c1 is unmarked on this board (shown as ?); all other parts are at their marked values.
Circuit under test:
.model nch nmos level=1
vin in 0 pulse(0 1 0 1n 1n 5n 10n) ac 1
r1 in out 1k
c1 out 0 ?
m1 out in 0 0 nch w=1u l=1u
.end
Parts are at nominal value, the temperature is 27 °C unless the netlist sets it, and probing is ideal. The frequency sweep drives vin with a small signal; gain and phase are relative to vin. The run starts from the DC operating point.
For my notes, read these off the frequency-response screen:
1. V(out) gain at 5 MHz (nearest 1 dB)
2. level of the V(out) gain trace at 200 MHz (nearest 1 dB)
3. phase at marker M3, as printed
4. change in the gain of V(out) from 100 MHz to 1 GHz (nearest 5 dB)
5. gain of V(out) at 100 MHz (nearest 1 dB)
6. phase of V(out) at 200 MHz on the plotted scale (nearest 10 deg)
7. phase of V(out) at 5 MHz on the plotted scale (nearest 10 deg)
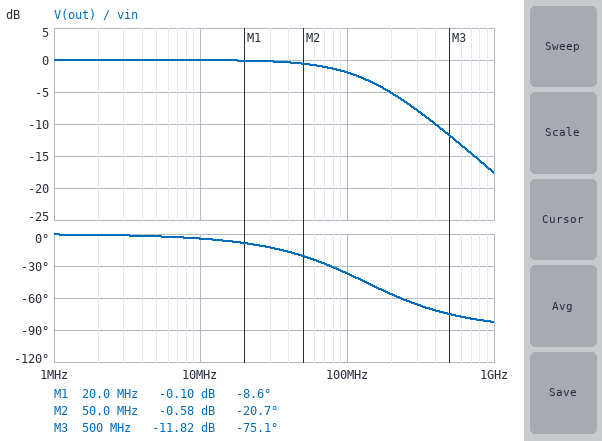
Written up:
0 dB
-5 dB
-75.1 deg
-15 dB
-2 dB
-60 deg
0 deg
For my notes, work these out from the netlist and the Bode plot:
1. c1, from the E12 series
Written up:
1.2 pF
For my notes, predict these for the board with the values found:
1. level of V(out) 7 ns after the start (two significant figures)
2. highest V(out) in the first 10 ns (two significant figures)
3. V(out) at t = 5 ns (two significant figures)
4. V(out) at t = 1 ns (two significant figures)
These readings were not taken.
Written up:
670 mV
980 mV
970 mV
320 mV
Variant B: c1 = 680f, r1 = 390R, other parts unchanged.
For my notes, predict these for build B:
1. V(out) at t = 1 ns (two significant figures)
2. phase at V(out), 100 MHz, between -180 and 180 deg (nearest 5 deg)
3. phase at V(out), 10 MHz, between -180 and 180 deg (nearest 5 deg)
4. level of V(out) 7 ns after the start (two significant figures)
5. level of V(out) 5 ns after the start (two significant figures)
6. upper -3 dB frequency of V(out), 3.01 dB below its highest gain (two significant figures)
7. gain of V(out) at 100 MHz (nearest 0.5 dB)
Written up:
740 mV
-10 deg
0 deg
260 mV
1.0 V
600 MHz
0 dB
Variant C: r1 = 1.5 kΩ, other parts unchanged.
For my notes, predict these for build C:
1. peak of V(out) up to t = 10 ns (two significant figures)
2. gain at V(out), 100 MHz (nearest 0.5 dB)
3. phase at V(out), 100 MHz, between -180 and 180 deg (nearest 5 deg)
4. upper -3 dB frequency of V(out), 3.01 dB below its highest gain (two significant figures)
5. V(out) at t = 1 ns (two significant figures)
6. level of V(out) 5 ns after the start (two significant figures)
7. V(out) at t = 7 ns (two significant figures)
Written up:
940 mV
-3.5 dB
-50 deg
88 MHz
230 mV
900 mV
730 mV
